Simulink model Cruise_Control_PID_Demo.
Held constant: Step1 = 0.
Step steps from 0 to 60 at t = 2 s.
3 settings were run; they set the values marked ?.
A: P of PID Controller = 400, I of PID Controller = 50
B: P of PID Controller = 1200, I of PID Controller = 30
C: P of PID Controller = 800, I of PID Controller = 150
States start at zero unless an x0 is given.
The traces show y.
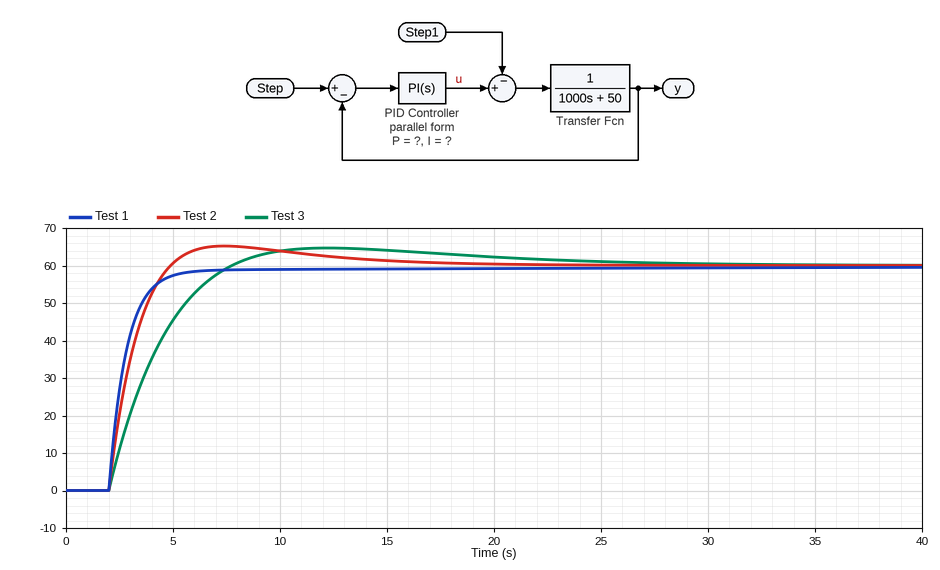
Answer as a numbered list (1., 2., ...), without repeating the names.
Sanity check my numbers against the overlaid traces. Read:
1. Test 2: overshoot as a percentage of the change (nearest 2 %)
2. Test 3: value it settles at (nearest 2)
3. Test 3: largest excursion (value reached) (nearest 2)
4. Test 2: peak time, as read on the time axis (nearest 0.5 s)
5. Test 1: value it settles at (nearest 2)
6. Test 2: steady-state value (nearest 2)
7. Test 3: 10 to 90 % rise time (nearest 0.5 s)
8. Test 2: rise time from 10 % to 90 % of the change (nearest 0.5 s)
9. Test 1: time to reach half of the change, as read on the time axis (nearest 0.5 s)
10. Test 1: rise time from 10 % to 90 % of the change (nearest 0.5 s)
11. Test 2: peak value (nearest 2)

1. 8 %
2. 60
3. 64
4. 7.5 s
5. 60
6. 60
7. 4.0 s
8. 2.0 s
9. 2.5 s
10. 2.0 s
11. 66
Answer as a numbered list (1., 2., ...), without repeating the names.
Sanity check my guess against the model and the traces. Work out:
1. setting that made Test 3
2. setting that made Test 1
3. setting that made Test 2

1. A
2. B
3. C
